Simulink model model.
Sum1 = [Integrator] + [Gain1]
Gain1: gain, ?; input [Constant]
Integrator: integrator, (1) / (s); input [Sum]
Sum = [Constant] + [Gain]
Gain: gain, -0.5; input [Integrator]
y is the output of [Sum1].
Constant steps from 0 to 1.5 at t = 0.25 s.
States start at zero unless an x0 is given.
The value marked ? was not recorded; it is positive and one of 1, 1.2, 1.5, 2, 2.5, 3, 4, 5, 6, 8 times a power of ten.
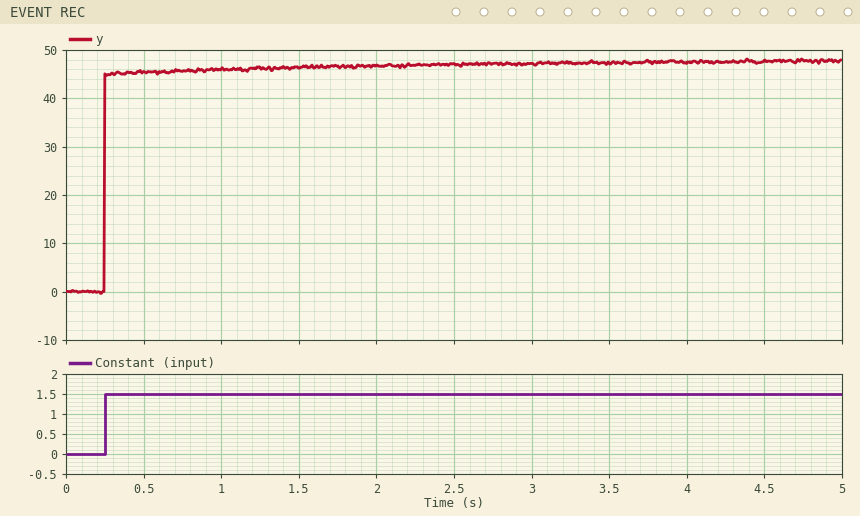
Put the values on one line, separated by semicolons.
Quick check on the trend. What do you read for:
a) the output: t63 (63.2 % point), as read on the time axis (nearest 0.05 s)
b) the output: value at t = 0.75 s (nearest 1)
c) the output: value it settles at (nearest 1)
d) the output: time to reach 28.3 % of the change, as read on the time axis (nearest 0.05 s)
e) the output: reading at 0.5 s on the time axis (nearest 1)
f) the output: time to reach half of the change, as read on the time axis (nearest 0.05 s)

0.25 s; 46; 48; 0.25 s; 45; 0.25 s
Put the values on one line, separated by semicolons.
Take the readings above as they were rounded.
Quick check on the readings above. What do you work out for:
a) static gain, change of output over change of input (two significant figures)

32
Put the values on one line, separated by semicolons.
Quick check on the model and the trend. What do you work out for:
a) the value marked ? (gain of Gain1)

30
